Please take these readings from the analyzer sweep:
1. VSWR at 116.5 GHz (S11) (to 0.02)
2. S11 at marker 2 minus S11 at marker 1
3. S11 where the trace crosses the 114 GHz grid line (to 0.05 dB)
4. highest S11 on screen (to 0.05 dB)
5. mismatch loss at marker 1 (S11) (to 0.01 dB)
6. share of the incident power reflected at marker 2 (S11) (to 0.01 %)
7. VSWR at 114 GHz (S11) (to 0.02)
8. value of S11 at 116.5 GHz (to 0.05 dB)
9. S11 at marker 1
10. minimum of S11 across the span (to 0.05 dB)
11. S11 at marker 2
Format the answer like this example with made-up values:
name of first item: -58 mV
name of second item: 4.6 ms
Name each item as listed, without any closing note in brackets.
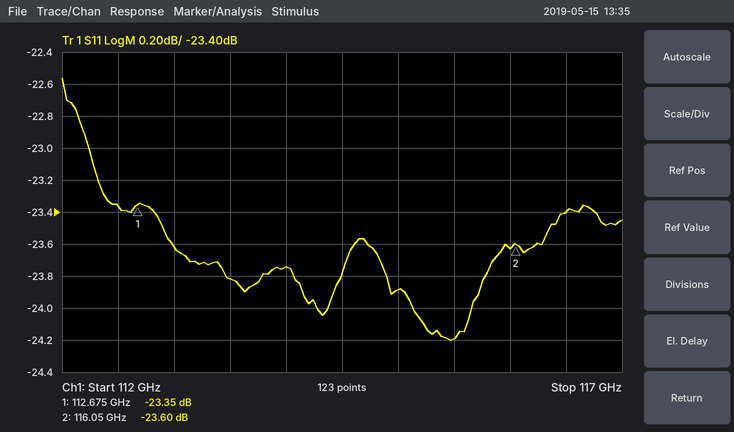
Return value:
VSWR at 116.5 GHz (S11): 1.14
S11 at marker 2 minus S11 at marker 1: -0.25 dB
S11 where the trace crosses the 114 GHz grid line: -23.75 dB
highest S11 on screen: -22.55 dB
mismatch loss at marker 1 (S11): 0.02 dB
share of the incident power reflected at marker 2 (S11): 0.44 %
VSWR at 114 GHz (S11): 1.14
value of S11 at 116.5 GHz: -23.40 dB
S11 at marker 1: -23.35 dB
minimum of S11 across the span: -24.20 dB
S11 at marker 2: -23.60 dB
